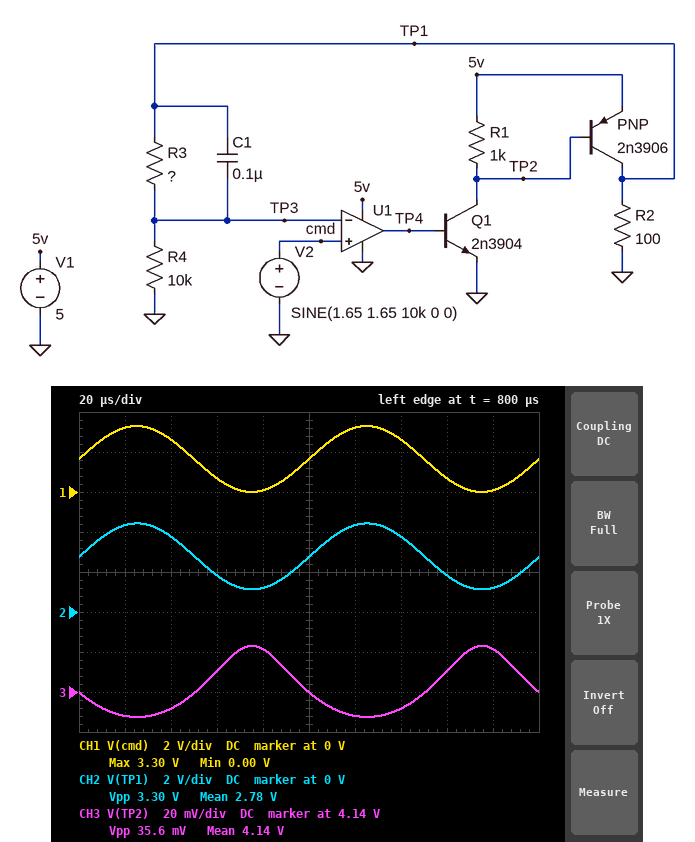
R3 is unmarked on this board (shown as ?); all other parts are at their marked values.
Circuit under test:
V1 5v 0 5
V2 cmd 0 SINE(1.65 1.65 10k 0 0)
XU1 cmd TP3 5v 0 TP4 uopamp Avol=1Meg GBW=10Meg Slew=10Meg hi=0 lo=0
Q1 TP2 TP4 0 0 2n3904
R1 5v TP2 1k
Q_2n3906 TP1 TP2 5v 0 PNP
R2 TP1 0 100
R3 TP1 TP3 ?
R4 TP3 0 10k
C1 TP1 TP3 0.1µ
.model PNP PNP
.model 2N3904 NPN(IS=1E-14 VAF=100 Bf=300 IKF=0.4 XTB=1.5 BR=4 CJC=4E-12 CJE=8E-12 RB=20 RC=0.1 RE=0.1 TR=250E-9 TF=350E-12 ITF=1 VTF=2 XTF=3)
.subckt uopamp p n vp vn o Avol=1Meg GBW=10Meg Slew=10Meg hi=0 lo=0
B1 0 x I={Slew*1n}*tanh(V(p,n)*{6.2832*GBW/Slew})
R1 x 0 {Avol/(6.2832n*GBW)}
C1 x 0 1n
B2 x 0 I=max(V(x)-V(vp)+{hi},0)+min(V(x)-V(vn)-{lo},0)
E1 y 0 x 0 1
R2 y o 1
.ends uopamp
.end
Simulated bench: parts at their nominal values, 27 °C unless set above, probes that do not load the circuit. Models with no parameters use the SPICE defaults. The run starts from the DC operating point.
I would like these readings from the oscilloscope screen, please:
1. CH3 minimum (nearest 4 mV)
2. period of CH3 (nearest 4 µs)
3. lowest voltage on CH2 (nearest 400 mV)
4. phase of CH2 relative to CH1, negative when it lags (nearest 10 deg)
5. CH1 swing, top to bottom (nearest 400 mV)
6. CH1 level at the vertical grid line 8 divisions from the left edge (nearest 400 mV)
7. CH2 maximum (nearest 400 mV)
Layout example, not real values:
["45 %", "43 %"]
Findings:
["4.128 V", "100 µs", "1.2 V", "0 deg", "3.2 V", "800 mV", "4.4 V"]
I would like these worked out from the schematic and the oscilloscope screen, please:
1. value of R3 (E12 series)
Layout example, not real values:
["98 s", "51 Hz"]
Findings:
["6.8 kΩ"]
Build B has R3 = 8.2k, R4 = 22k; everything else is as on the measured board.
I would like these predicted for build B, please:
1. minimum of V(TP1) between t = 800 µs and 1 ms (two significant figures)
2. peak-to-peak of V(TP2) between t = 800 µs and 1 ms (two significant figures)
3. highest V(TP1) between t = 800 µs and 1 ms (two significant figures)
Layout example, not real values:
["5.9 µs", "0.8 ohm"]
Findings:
["620 mV", "48 mV", "3.9 V"]
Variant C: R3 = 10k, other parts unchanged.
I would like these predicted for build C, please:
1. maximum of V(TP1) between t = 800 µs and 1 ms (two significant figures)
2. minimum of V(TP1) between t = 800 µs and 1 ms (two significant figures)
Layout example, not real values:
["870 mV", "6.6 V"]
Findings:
["5.0 V", "1.7 V"]
